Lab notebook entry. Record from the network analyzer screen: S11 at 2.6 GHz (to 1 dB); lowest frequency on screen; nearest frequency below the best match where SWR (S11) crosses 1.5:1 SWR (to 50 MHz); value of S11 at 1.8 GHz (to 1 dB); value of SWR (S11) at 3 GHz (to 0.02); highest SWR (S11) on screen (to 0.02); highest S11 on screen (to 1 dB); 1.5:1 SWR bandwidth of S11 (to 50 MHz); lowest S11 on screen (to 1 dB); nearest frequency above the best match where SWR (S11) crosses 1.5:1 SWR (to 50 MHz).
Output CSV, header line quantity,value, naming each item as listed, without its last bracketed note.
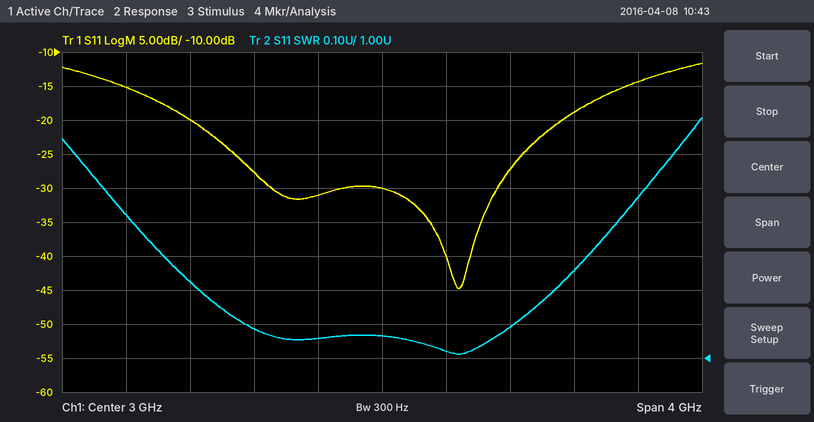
quantity,value
S11 at 2.6 GHz,-31 dB
lowest frequency on screen,1 GHz
nearest frequency below the best match where SWR (S11) crosses 1.5:1 SWR,1.25 GHz
value of S11 at 1.8 GHz,-20 dB
value of SWR (S11) at 3 GHz,1.06
highest SWR (S11) on screen,1.70
highest S11 on screen,-12 dB
1.5:1 SWR bandwidth of S11,3.40 GHz
lowest S11 on screen,-45 dB
nearest frequency above the best match where SWR (S11) crosses 1.5:1 SWR,4.65 GHz
